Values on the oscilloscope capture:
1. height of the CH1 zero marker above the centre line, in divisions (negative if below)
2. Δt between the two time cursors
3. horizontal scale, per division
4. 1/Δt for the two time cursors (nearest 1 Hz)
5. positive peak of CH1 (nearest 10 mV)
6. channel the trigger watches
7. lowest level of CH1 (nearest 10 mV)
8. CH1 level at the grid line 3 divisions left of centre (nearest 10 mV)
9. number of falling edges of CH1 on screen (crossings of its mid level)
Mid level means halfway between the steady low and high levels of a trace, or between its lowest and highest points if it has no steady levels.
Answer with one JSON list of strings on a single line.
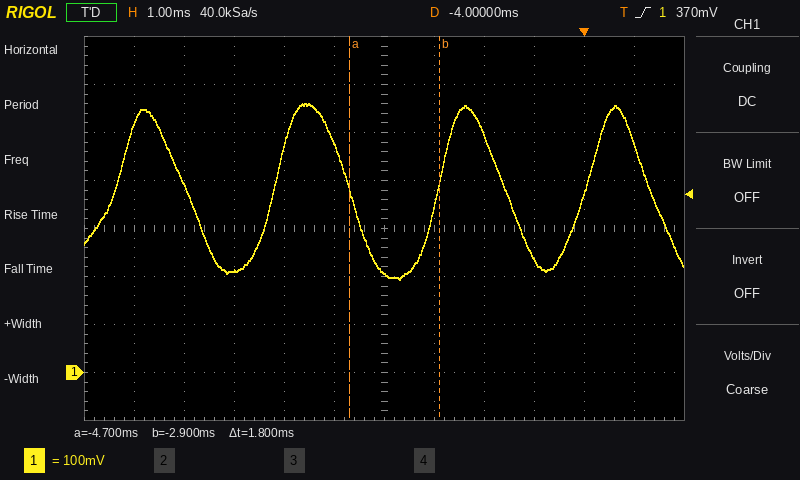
["-3.0 div", "1.8 ms", "1 ms", "556 Hz", "560 mV", "CH1", "190 mV", "210 mV", "4"]
